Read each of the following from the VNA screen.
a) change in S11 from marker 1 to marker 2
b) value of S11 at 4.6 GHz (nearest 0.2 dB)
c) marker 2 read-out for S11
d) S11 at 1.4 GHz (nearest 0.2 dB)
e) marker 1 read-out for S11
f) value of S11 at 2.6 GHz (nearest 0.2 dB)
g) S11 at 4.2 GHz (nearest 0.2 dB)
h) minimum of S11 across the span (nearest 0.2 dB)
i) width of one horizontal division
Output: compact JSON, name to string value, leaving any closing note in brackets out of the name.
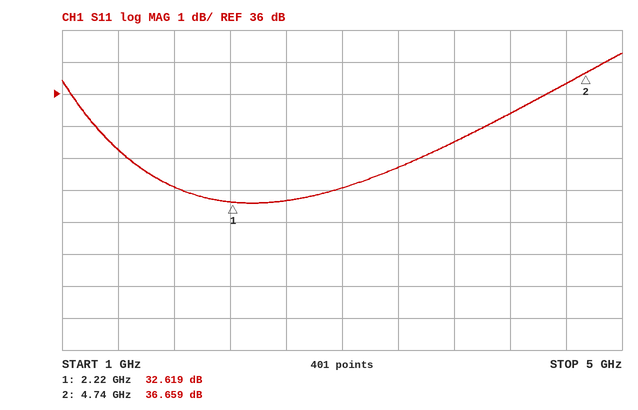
{"change in S11 from marker 1 to marker 2": "4.040 dB", "value of S11 at 4.6 GHz": "36.4 dB", "marker 2 read-out for S11": "36.659 dB", "S11 at 1.4 GHz": "34.2 dB", "marker 1 read-out for S11": "32.619 dB", "value of S11 at 2.6 GHz": "32.6 dB", "S11 at 4.2 GHz": "35.4 dB", "minimum of S11 across the span": "32.6 dB", "width of one horizontal division": "400 MHz"}
